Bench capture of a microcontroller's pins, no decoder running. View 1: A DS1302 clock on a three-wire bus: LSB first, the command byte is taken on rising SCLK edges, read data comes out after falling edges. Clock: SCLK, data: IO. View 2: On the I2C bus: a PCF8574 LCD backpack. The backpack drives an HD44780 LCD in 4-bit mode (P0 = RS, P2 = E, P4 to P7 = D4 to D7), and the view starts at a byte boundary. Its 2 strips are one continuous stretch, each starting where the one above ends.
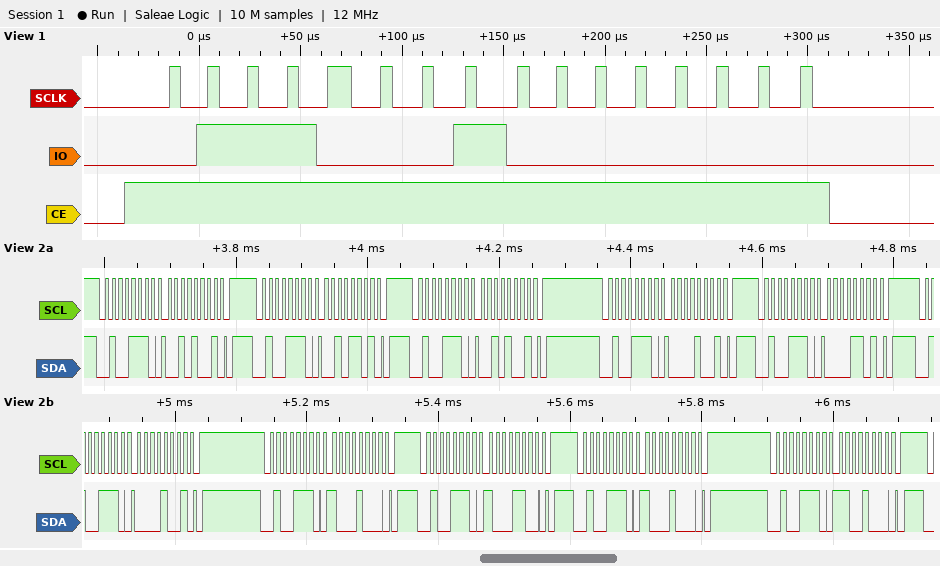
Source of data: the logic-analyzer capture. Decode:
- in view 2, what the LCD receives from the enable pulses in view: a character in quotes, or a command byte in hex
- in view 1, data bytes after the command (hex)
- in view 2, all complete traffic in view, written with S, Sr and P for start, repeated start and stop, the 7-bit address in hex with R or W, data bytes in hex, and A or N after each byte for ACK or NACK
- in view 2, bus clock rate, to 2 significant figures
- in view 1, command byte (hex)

' '
00
S 27W A 29 A P S 27W A 2D A P S 27W A 29 A P S 27W A 09 A P S 27W A 0D A P S 27W A 09 A P S 27W A 88 A P S 27W A 8C A P S 27W A 88 A P S 27W A C8 A P
100 kHz
0x8E
